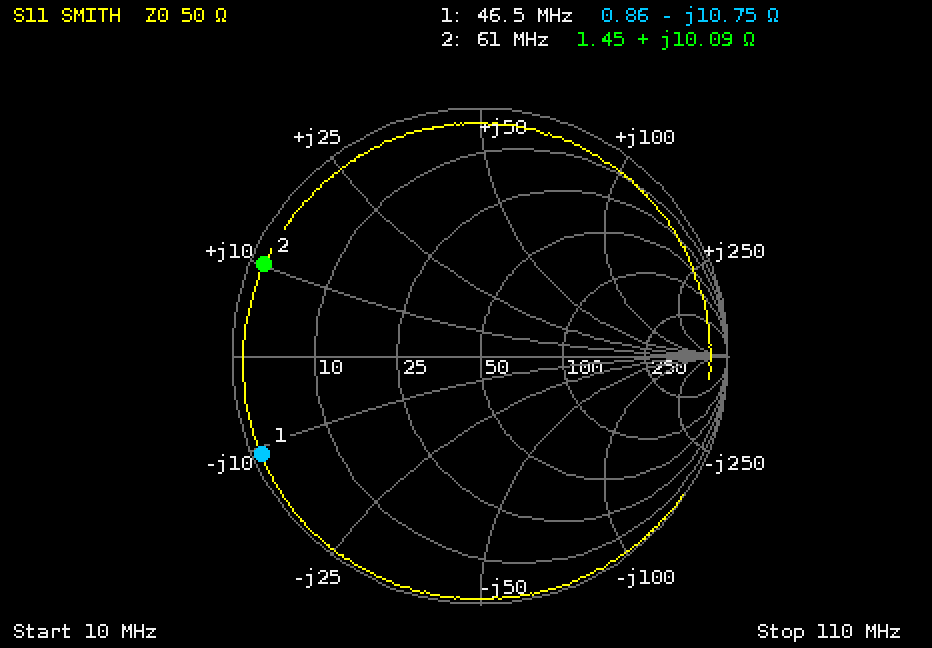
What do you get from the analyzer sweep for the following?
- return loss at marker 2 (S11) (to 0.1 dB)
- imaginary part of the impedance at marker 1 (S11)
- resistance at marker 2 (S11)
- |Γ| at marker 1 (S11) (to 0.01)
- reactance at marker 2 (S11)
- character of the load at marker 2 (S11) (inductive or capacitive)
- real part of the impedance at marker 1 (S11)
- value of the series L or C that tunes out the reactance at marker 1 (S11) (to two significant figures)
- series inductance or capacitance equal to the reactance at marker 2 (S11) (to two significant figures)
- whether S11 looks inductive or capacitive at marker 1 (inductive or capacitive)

0.5 dB
-10.75 Ω
1.45 Ω
0.97
+10.09 Ω
inductive
0.86 Ω
37 nH
26 nH
capacitive
